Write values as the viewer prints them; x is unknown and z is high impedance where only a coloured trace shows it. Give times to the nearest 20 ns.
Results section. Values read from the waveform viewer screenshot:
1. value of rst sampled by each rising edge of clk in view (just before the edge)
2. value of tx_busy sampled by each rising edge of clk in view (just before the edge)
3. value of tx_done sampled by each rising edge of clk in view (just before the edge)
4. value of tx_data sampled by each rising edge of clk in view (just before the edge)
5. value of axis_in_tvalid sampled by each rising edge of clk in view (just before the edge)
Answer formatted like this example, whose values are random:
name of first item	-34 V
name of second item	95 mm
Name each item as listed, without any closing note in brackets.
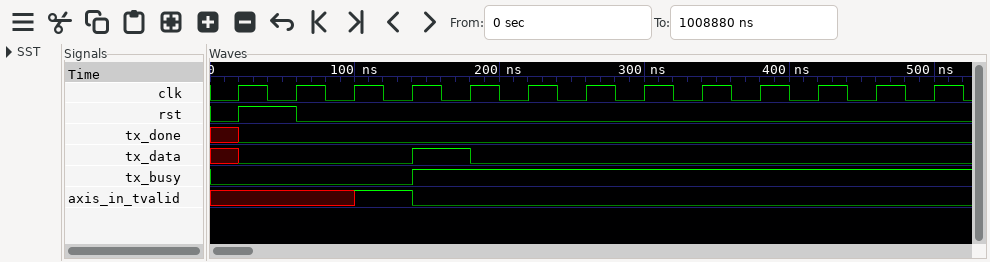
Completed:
value of rst sampled by each rising edge of clk in view	0 1 0 0 0 0 0 0 0 0 0 0 0
value of tx_busy sampled by each rising edge of clk in view	0 0 0 0 1 1 1 1 1 1 1 1 1
value of tx_done sampled by each rising edge of clk in view	x 0 0 0 0 0 0 0 0 0 0 0 0
value of tx_data sampled by each rising edge of clk in view	x 0 0 0 1 0 0 0 0 0 0 0 0
value of axis_in_tvalid sampled by each rising edge of clk in view	x x x 1 0 0 0 0 0 0 0 0 0
